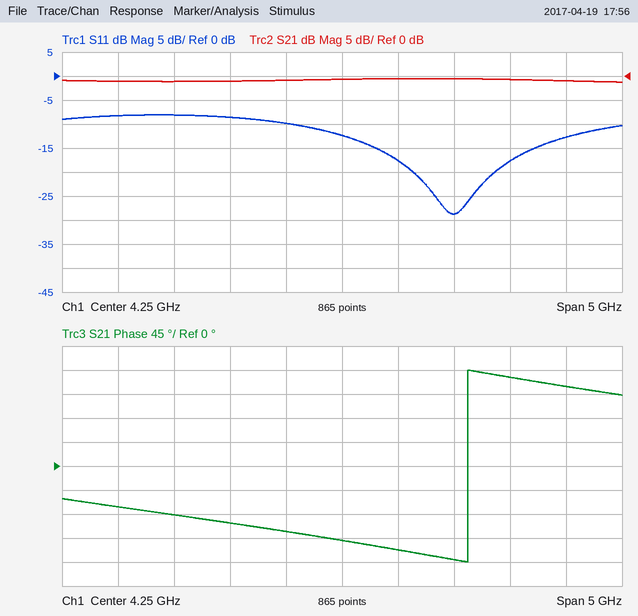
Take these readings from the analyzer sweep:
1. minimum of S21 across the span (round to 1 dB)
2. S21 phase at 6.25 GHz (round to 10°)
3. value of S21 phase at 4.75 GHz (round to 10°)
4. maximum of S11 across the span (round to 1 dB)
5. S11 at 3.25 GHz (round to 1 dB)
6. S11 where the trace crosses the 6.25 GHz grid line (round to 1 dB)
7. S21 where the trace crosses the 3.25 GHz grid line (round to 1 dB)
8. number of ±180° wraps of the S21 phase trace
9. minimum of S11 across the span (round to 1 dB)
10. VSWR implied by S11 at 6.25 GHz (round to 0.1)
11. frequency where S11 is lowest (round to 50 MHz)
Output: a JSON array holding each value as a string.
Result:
["-1 dB", "150°", "-160°", "-8 dB", "-9 dB", "-13 dB", "-1 dB", "1", "-29 dB", "1.6", "5.25 GHz"]
